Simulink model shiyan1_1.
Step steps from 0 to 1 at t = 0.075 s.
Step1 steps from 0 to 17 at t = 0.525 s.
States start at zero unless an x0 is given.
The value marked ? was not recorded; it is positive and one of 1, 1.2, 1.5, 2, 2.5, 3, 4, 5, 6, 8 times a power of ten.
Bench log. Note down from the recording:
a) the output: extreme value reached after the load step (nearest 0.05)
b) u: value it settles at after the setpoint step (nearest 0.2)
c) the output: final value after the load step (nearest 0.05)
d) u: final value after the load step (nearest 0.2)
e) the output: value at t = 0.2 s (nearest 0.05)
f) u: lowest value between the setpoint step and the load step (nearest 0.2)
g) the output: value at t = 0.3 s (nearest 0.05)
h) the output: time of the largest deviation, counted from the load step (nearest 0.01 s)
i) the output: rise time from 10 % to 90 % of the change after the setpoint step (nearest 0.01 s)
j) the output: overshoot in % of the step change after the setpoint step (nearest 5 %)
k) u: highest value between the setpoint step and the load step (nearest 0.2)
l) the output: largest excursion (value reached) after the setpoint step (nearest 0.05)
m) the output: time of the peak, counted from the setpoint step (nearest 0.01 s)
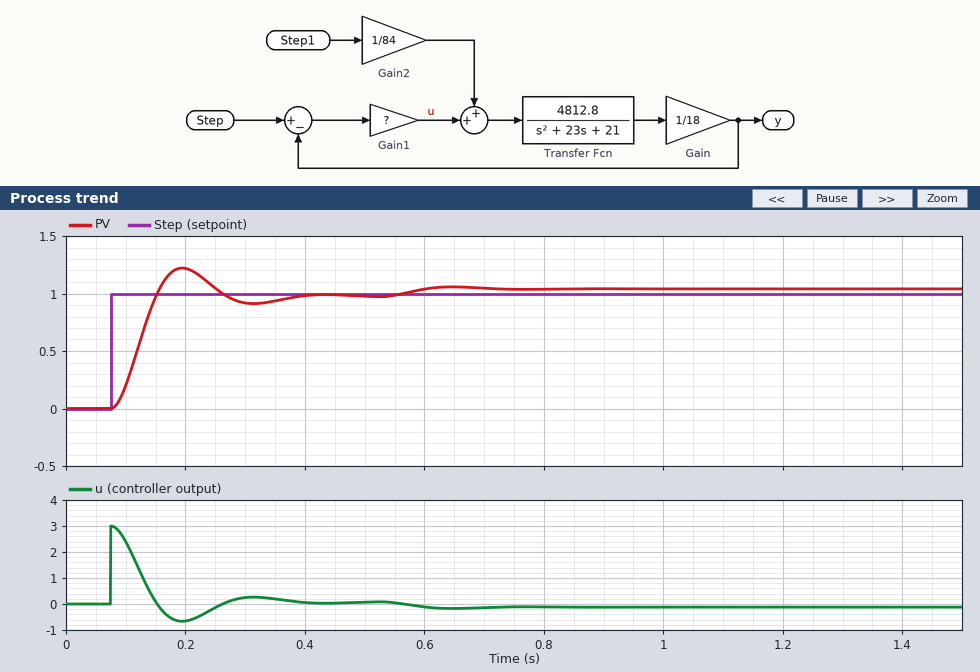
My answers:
1.05
0.0
1.05
-0.2
1.20
-0.6
0.90
0.12 s
0.05 s
25 %
3.0
1.20
0.12 s
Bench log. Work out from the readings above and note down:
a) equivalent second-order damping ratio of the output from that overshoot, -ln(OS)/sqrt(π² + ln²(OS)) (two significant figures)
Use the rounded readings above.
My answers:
0.40
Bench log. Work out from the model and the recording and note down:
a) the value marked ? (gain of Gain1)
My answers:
3
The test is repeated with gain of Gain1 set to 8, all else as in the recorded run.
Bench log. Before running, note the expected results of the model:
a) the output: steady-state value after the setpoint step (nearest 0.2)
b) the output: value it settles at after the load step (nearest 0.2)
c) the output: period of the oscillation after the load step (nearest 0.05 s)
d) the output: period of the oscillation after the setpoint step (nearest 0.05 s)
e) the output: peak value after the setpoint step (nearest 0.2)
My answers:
1.0
1.0
0.15 s
0.15 s
1.4
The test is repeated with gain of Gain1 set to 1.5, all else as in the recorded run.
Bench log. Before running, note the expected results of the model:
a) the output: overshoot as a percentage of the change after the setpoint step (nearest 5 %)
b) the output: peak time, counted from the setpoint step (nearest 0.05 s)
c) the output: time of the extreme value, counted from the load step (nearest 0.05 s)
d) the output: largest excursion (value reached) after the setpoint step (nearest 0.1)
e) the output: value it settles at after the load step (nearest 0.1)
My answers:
10 %
0.20 s
0.20 s
1.1
1.1
